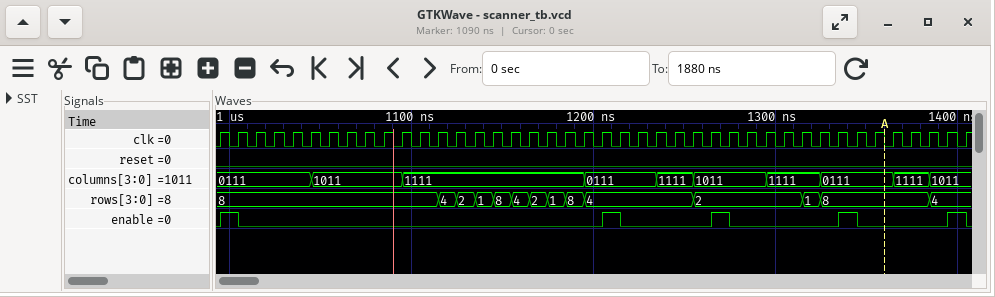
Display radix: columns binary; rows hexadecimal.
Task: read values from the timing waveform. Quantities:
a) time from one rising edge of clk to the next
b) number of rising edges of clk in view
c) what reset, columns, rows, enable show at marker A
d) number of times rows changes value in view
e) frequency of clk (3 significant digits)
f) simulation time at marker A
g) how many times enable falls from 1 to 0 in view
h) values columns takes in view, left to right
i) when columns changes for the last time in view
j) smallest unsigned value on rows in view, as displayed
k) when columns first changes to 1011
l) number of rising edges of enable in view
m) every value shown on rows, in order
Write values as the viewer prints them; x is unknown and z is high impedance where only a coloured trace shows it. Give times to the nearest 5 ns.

10 ns
42
reset=0, columns=0111, rows=8, enable=0
13
100 MHz
1360 ns
5
0111, 1011, 1111, 0111, 1111, 1011, 1111, 0111, 1111, 1011
1385 ns
1
1045 ns
5
8, 4, 2, 1, 8, 4, 2, 1, 8, 4, 2, 1, 8, 4
